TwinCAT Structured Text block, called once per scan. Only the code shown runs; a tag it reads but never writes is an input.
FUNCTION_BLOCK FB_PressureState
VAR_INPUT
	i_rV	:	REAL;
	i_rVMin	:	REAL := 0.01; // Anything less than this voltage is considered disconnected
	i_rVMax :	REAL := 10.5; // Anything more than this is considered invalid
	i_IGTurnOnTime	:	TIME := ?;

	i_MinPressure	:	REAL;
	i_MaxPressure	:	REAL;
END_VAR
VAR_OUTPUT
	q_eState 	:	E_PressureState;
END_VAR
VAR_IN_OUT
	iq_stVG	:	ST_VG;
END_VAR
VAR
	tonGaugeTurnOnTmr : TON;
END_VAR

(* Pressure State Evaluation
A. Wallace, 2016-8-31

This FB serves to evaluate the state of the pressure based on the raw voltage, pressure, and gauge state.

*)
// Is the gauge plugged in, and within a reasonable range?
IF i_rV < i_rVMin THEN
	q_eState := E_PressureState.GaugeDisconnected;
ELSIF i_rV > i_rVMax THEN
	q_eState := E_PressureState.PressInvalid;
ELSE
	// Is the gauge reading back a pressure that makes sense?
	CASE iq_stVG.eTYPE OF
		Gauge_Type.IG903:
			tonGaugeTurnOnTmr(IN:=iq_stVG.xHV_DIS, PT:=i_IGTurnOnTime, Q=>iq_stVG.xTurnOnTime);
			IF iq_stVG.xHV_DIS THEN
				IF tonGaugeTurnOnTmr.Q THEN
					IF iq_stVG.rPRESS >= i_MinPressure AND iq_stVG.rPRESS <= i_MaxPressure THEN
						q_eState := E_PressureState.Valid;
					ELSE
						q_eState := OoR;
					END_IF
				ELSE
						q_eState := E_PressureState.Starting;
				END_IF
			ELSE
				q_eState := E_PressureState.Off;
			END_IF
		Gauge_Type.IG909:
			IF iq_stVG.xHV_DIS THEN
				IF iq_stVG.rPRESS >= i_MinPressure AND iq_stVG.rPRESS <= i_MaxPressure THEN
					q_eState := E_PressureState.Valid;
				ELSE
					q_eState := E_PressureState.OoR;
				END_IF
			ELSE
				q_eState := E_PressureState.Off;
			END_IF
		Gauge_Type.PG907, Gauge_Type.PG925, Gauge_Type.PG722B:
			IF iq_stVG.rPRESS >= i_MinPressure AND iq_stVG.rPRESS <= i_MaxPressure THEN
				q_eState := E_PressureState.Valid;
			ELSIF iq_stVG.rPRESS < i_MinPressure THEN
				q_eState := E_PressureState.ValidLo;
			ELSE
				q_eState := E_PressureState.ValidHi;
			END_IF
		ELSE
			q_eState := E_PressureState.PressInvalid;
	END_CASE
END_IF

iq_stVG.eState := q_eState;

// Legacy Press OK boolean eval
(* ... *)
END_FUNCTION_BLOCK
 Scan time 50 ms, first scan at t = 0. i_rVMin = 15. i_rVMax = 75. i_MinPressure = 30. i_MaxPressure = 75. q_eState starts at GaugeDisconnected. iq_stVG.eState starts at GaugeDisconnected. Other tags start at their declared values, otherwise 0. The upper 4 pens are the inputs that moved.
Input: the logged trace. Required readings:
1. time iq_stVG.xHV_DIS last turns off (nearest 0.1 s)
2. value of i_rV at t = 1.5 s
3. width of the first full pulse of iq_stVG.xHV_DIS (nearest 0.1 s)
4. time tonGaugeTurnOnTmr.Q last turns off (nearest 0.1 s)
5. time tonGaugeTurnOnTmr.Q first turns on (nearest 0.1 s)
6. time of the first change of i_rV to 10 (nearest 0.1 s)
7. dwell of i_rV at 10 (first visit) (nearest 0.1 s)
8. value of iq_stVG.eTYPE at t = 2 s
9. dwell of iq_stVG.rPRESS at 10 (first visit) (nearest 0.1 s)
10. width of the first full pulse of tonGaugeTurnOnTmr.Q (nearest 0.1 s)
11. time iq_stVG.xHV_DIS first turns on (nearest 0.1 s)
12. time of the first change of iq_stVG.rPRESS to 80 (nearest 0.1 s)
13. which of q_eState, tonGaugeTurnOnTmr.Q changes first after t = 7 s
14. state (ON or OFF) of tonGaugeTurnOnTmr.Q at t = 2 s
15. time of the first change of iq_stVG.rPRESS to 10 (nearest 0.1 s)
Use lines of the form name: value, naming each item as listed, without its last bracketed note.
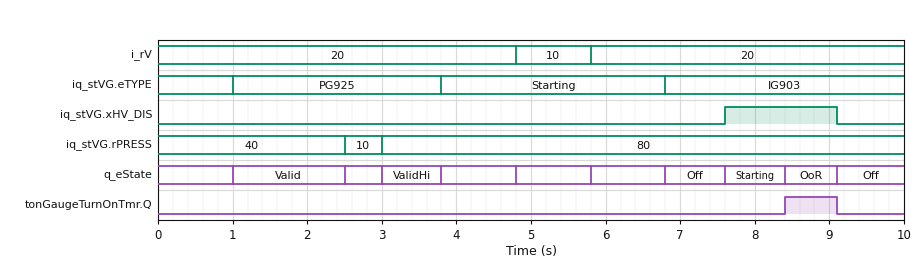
time iq_stVG.xHV_DIS last turns off: 9.1 s
value of i_rV at t = 1.5 s: 20
width of the first full pulse of iq_stVG.xHV_DIS: 1.5 s
time tonGaugeTurnOnTmr.Q last turns off: 9.1 s
time tonGaugeTurnOnTmr.Q first turns on: 8.4 s
time of the first change of i_rV to 10: 4.8 s
dwell of i_rV at 10 (first visit): 1.0 s
value of iq_stVG.eTYPE at t = 2 s: PG925
dwell of iq_stVG.rPRESS at 10 (first visit): 0.5 s
width of the first full pulse of tonGaugeTurnOnTmr.Q: 0.7 s
time iq_stVG.xHV_DIS first turns on: 7.6 s
time of the first change of iq_stVG.rPRESS to 80: 3.0 s
which of q_eState, tonGaugeTurnOnTmr.Q changes first after t = 7 s: q_eState
state (ON or OFF) of tonGaugeTurnOnTmr.Q at t = 2 s: OFF
time of the first change of iq_stVG.rPRESS to 10: 2.5 s
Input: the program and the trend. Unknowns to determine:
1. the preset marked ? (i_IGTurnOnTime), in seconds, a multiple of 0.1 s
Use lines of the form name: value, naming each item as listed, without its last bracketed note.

the preset marked ? (i_IGTurnOnTime), in seconds, a multiple of 0.1 s: 0.8 s
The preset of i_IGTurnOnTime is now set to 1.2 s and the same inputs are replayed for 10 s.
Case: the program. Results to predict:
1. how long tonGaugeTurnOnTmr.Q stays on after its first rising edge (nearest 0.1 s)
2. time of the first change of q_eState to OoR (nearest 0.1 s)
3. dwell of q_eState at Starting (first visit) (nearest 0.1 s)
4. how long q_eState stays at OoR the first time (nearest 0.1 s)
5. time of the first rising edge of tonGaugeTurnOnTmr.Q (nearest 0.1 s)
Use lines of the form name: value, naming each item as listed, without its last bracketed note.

how long tonGaugeTurnOnTmr.Q stays on after its first rising edge: 0.3 s
time of the first change of q_eState to OoR: 8.8 s
dwell of q_eState at Starting (first visit): 1.2 s
how long q_eState stays at OoR the first time: 0.3 s
time of the first rising edge of tonGaugeTurnOnTmr.Q: 8.8 s
